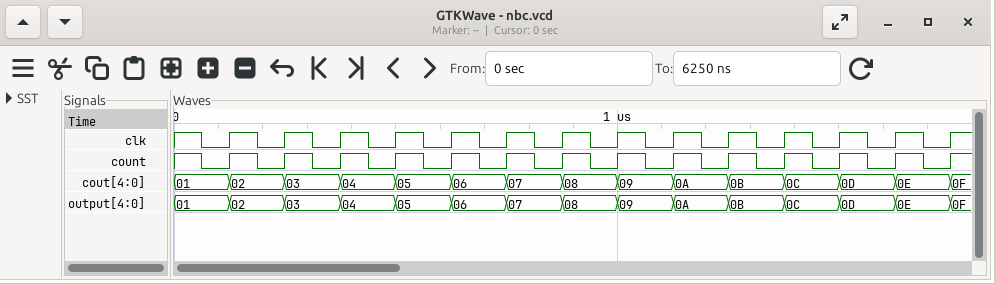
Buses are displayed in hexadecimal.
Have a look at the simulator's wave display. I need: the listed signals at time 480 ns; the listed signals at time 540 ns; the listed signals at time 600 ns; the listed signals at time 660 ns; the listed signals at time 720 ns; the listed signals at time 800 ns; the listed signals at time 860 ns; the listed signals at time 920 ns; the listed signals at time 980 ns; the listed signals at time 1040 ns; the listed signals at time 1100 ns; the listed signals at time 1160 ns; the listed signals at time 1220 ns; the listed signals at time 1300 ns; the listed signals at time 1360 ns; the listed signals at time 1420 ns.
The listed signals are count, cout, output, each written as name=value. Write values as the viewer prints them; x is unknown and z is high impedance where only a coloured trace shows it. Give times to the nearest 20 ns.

count=0, cout=04, output=04
count=1, cout=05, output=05
count=0, cout=05, output=05
count=1, cout=06, output=06
count=0, cout=06, output=06
count=1, cout=07, output=07
count=0, cout=07, output=07
count=1, cout=08, output=08
count=0, cout=08, output=08
count=1, cout=09, output=09
count=0, cout=09, output=09
count=1, cout=0A, output=0A
count=0, cout=0A, output=0A
count=1, cout=0B, output=0B
count=0, cout=0B, output=0B
count=1, cout=0C, output=0C
